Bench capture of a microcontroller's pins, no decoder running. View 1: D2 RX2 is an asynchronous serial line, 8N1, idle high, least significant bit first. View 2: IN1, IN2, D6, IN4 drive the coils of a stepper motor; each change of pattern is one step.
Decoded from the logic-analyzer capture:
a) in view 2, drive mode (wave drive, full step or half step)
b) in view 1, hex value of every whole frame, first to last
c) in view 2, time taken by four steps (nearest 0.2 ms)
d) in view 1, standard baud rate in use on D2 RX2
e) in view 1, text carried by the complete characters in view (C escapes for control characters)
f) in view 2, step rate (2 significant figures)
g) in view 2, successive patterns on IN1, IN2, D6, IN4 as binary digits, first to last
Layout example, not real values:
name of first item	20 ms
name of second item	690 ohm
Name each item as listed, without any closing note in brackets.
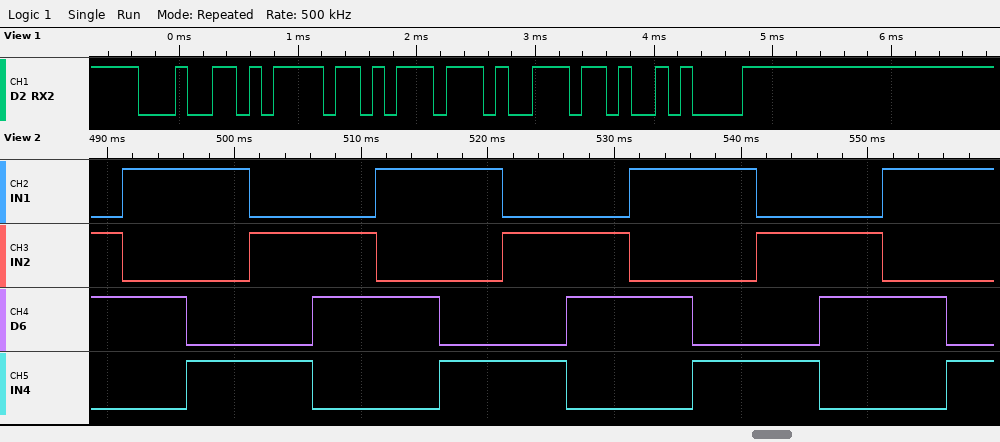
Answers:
in view 2, drive mode	full step
in view 1, hex value of every whole frame, first to last	64 6F 77 6E 0A
in view 2, time taken by four steps	20.0 ms
in view 1, standard baud rate in use on D2 RX2	9600 baud
in view 1, text carried by the complete characters in view	"down\n"
in view 2, step rate	200 steps/s
in view 2, successive patterns on IN1, IN2, D6, IN4 as binary digits, first to last	0110 1010 1001 0101 0110 1010 1001 0101 0110 1010 1001 0101 0110 1010 1001
